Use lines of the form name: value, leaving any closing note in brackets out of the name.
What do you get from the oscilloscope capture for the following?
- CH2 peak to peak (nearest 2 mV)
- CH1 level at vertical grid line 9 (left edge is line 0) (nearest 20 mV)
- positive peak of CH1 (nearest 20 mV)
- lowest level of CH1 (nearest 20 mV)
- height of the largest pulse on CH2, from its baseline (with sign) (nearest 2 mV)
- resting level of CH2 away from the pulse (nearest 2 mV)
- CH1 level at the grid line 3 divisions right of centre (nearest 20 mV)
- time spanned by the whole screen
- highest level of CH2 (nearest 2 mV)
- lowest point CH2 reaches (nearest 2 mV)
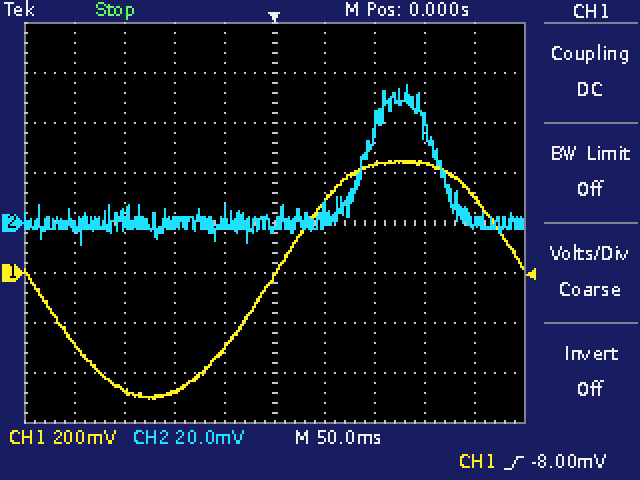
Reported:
CH2 peak to peak: 64 mV
CH1 level at vertical grid line 9 (left edge is line 0): 300 mV
positive peak of CH1: 440 mV
lowest level of CH1: -500 mV
height of the largest pulse on CH2, from its baseline (with sign): +56 mV
resting level of CH2 away from the pulse: 0 mV
CH1 level at the grid line 3 divisions right of centre: 440 mV
time spanned by the whole screen: 500 ms
highest level of CH2: 56 mV
lowest point CH2 reaches: -8 mV
